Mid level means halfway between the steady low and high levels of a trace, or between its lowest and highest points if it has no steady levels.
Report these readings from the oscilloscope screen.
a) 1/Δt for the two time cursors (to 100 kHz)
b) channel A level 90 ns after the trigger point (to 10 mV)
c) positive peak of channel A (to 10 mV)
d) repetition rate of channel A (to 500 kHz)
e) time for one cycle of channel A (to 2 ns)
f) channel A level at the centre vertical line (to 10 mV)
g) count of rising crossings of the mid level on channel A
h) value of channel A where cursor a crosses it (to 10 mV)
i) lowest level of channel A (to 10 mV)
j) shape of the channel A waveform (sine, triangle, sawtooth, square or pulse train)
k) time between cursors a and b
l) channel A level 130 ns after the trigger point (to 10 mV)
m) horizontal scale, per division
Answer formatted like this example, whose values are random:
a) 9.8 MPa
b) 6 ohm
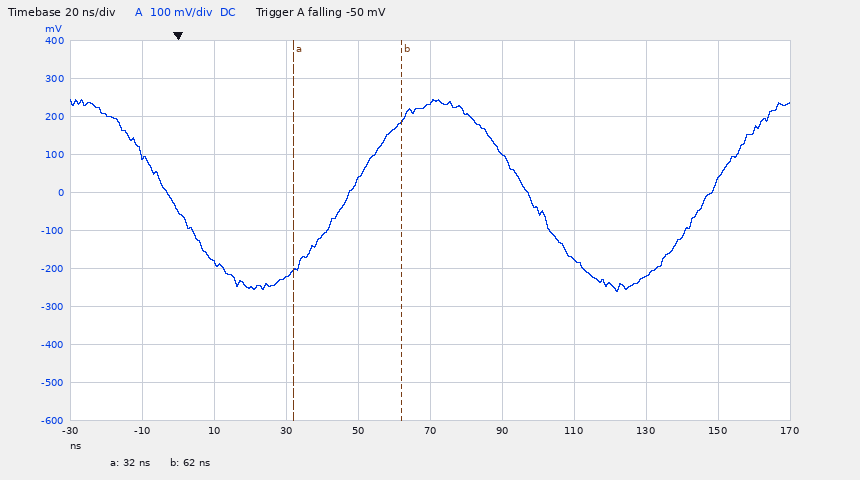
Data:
a) 33.3 MHz
b) 100 mV
c) 240 mV
d) 10.0 MHz
e) 100 ns
f) 240 mV
g) 2
h) -210 mV
i) -260 mV
j) sine
k) 30 ns
l) -220 mV
m) 20 ns
